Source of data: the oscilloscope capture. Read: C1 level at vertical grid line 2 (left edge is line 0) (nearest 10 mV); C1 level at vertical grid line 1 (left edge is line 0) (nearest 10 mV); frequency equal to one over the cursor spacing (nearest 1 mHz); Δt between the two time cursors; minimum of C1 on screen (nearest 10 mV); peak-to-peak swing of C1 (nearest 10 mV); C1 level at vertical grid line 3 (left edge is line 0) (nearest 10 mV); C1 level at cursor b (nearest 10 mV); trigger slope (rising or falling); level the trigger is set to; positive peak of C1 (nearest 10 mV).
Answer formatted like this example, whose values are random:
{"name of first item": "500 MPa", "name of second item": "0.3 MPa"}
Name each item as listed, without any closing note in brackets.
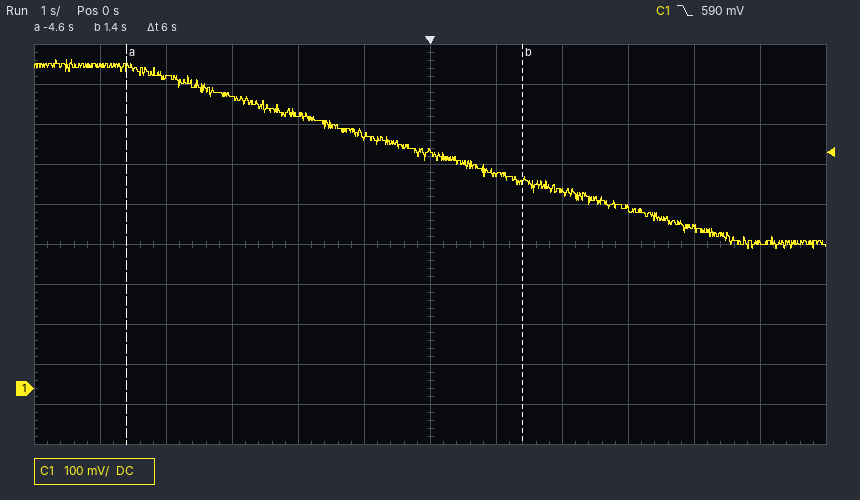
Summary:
{"C1 level at vertical grid line 2 (left edge is line 0)": "780 mV", "C1 level at vertical grid line 1 (left edge is line 0)": "810 mV", "frequency equal to one over the cursor spacing": "167 mHz", "Δt between the two time cursors": "6 s", "minimum of C1 on screen": "350 mV", "peak-to-peak swing of C1": "470 mV", "C1 level at vertical grid line 3 (left edge is line 0)": "730 mV", "C1 level at cursor b": "520 mV", "trigger slope": "falling", "level the trigger is set to": "590 mV", "positive peak of C1": "820 mV"}
